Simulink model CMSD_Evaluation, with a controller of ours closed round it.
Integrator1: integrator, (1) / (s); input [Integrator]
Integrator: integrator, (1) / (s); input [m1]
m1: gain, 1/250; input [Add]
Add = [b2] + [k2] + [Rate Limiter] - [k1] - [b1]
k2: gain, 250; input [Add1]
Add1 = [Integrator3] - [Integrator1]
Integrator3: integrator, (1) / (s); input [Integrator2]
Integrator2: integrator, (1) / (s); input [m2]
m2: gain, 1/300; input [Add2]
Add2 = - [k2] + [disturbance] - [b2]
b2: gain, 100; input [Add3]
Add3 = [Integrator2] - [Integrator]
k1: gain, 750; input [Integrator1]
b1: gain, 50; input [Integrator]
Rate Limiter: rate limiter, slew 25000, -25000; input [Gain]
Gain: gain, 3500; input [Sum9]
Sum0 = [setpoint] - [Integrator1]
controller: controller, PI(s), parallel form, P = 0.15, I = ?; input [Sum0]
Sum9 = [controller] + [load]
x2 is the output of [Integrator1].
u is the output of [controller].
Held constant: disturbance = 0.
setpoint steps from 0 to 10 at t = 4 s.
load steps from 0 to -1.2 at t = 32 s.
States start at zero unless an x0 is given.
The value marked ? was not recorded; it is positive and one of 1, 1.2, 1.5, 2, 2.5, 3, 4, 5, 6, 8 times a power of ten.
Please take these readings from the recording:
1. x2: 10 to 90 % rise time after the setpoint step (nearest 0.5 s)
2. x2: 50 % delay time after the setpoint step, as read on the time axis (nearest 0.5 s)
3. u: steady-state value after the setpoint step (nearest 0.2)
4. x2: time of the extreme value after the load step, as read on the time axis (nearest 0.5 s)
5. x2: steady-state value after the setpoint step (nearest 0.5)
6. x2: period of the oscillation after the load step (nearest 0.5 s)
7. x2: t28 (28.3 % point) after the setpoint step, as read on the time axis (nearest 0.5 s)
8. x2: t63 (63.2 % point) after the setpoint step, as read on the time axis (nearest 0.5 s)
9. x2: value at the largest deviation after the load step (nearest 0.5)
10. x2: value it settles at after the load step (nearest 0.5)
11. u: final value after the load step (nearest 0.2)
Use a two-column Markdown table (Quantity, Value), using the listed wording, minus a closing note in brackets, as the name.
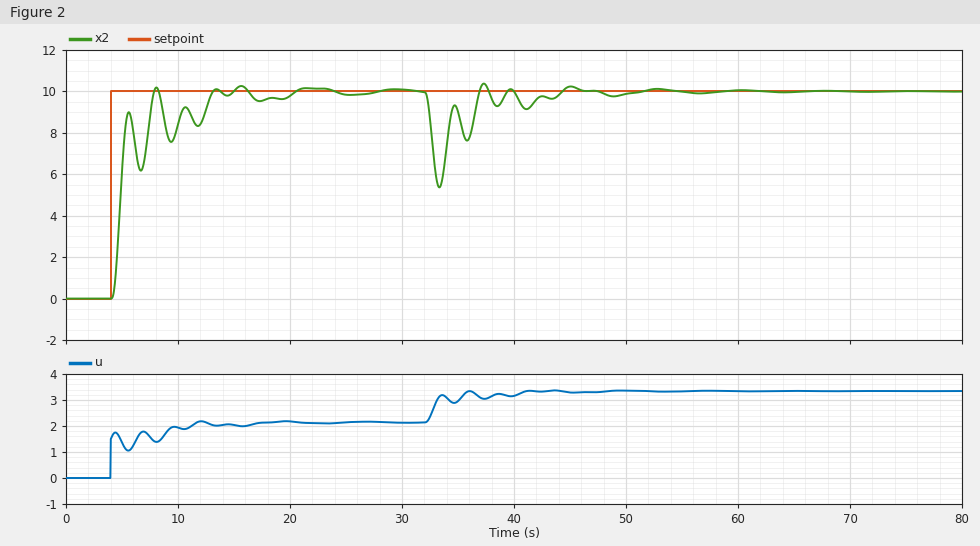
| Quantity | Value |
|---|---|
| x2: 10 to 90 % rise time after the setpoint step | 3.0 s |
| x2: 50 % delay time after the setpoint step, as read on the time axis | 5.0 s |
| u: steady-state value after the setpoint step | 2.2 |
| x2: time of the extreme value after the load step, as read on the time axis | 33.5 s |
| x2: steady-state value after the setpoint step | 10.0 |
| x2: period of the oscillation after the load step | 2.5 s |
| x2: t28 (28.3 % point) after the setpoint step, as read on the time axis | 4.5 s |
| x2: t63 (63.2 % point) after the setpoint step, as read on the time axis | 5.0 s |
| x2: value at the largest deviation after the load step | 5.5 |
| x2: value it settles at after the load step | 10.0 |
| u: final value after the load step | 3.4 |
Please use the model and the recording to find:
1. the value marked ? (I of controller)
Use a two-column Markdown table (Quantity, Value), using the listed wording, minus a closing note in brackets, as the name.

| Quantity | Value |
|---|---|
| the value marked ? | 0.1 |
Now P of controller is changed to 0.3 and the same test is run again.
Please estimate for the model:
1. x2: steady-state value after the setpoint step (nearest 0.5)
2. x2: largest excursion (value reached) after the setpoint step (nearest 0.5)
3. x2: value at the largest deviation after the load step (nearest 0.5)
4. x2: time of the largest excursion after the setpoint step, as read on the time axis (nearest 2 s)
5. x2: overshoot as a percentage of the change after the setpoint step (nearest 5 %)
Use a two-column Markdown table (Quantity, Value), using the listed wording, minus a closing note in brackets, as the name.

| Quantity | Value |
|---|---|
| x2: steady-state value after the setpoint step | 10.0 |
| x2: largest excursion (value reached) after the setpoint step | 11.0 |
| x2: value at the largest deviation after the load step | 6.5 |
| x2: time of the largest excursion after the setpoint step, as read on the time axis | 8 s |
| x2: overshoot as a percentage of the change after the setpoint step | 10 % |
